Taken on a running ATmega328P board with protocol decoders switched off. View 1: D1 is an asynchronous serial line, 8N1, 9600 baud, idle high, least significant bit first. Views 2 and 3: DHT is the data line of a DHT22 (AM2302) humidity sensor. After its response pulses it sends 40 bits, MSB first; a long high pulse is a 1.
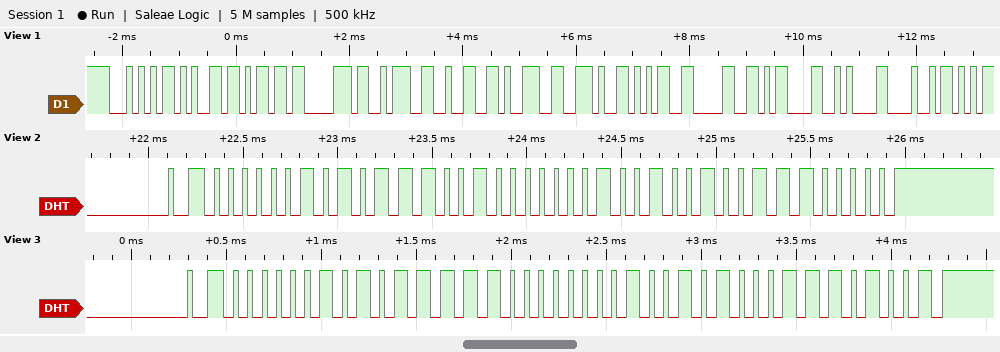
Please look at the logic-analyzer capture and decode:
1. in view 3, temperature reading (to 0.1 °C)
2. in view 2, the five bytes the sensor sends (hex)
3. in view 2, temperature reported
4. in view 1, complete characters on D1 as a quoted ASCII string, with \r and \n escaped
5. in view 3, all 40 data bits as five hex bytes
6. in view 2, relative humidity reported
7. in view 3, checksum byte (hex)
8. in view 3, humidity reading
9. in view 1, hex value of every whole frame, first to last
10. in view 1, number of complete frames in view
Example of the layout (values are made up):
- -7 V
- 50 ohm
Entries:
- 29.6 °C
- 02 B9 01 24 E0
- 29.2 °C
- "Temp:29.50\r\nH"
- 02 BE 01 28 E9
- 69.7 %
- 0xE9
- 70.2 %
- 54 65 6D 70 3A 32 39 2E 35 30 0D 0A 48
- 13
